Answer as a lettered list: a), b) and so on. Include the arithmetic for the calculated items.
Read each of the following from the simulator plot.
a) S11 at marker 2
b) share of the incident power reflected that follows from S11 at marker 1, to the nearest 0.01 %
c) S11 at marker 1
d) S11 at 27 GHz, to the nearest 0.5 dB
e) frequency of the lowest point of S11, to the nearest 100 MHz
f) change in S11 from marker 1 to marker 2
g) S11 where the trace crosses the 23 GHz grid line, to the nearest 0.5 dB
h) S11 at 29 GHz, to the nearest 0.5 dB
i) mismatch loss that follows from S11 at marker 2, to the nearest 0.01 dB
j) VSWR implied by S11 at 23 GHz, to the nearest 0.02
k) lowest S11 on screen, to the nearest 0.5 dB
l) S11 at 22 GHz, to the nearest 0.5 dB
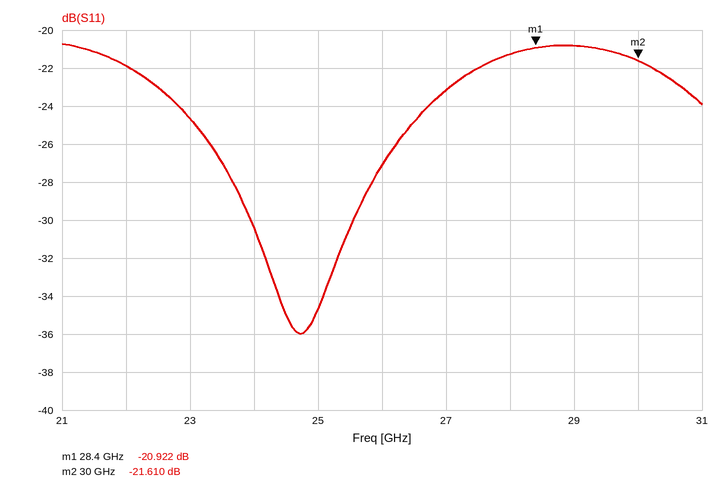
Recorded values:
a) -21.610 dB
b) 10^(-20.922/10) ≈ 0.81 %
c) -20.922 dB
d) -23.0 dB
e) 24.7 GHz
f) -21.61 − (-20.922) = -0.688 dB
g) -24.5 dB
h) -21.0 dB
i) −10 log10(1 − 10^(-21.61/10)) ≈ 0.03 dB
j) |Γ| = 10^(-24.5/20) = 0.0596; VSWR = (1 + 0.0596)/(1 − 0.0596) ≈ 1.13, so 1.12 to the nearest 0.02
k) -36.0 dB
l) -22.0 dB
